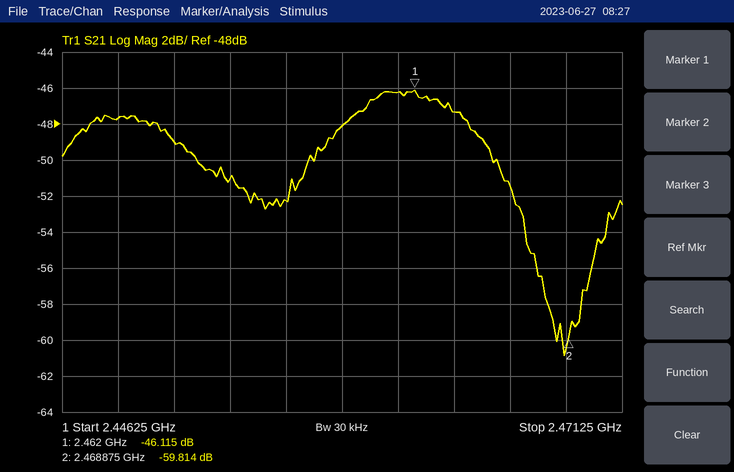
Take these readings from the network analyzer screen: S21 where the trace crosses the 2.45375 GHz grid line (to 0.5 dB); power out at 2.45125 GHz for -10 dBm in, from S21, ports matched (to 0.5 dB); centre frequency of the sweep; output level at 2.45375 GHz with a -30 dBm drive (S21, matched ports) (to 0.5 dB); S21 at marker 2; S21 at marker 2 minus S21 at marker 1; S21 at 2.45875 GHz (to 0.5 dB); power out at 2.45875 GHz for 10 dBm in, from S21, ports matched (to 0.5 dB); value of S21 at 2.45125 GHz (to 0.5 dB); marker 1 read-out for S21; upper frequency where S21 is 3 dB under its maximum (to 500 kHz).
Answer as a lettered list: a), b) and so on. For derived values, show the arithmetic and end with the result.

a) -51.0 dB
b) -10 dBm + (-49.0 dB) = -59.0 dBm
c) 2.45875 GHz
d) -30 dBm + (-51.0 dB) = -81.0 dBm
e) -59.814 dB
f) -59.814 − (-46.115) = -13.699 dB
g) -48.0 dB
h) 10 dBm + (-48.0 dB) = -38.0 dBm
i) -49.0 dB
j) -46.115 dB
k) 2.4650 GHz
